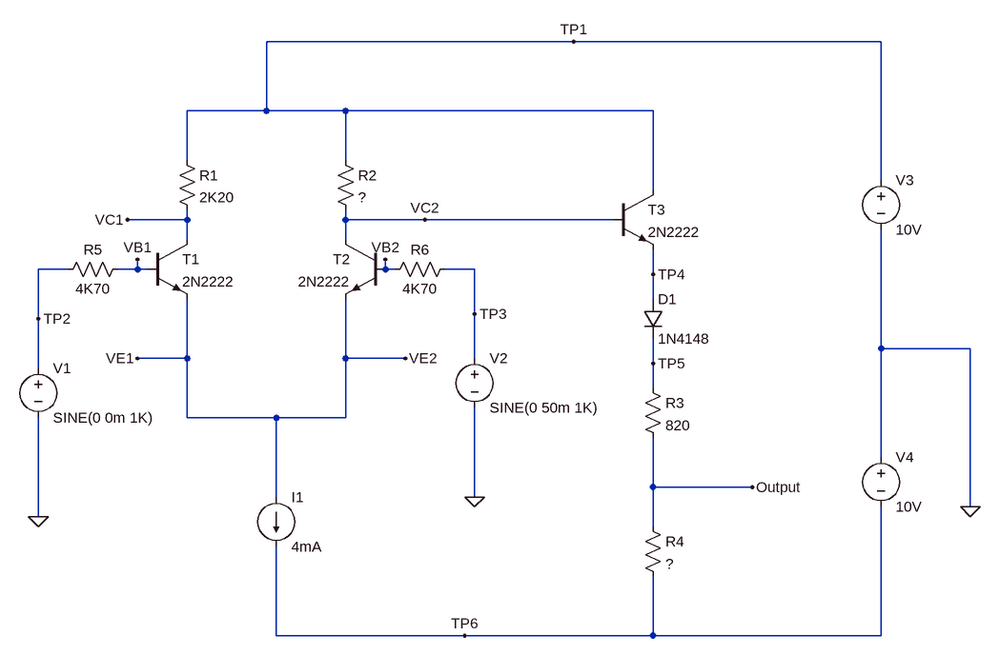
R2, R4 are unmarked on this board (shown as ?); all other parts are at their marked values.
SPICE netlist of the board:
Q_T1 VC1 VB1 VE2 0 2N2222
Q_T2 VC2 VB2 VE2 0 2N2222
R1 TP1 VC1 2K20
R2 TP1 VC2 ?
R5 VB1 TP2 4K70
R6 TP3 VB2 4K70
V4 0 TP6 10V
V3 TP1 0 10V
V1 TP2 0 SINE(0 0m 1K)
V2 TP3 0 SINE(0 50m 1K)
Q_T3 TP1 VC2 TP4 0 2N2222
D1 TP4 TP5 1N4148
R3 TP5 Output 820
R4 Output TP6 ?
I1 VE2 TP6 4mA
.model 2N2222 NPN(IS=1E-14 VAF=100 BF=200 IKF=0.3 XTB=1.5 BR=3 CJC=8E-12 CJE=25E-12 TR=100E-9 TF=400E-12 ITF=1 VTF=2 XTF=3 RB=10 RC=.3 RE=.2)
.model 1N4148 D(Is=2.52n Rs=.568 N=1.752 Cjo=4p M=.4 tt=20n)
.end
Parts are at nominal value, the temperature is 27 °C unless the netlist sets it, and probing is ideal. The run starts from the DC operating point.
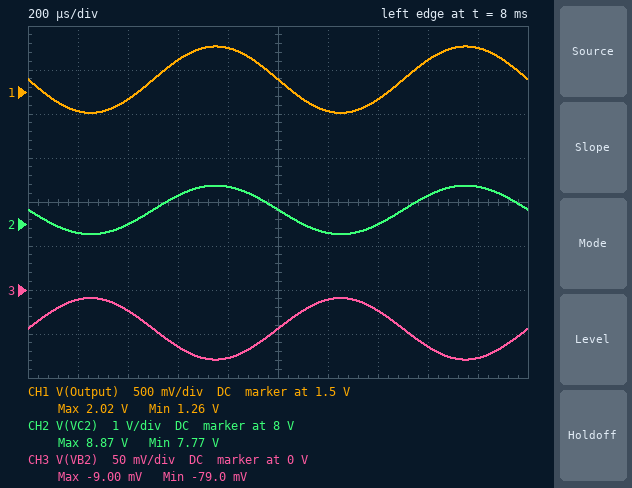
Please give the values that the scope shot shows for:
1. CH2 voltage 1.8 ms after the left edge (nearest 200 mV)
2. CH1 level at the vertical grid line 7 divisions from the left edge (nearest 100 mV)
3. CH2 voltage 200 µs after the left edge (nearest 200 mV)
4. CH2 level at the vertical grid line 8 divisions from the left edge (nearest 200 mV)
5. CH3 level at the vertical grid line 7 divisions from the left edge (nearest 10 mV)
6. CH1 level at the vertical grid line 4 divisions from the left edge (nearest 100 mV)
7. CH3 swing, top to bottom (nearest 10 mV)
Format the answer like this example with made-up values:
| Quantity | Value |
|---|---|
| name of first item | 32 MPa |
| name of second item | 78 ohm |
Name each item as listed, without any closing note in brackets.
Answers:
| Quantity | Value |
|---|---|
| CH2 voltage 1.8 ms after the left edge | 8.8 V |
| CH1 level at the vertical grid line 7 divisions from the left edge | 1.4 V |
| CH2 voltage 200 µs after the left edge | 7.8 V |
| CH2 level at the vertical grid line 8 divisions from the left edge | 8.6 V |
| CH3 level at the vertical grid line 7 divisions from the left edge | -20 mV |
| CH1 level at the vertical grid line 4 divisions from the left edge | 2.0 V |
| CH3 swing, top to bottom | 70 mV |
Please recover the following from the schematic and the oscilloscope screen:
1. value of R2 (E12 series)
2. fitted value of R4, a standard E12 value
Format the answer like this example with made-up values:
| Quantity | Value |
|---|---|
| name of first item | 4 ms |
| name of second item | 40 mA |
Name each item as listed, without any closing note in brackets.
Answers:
| Quantity | Value |
|---|---|
| value of R2 | 820 Ω |
| fitted value of R4, a standard E12 value | 1.8 kΩ |
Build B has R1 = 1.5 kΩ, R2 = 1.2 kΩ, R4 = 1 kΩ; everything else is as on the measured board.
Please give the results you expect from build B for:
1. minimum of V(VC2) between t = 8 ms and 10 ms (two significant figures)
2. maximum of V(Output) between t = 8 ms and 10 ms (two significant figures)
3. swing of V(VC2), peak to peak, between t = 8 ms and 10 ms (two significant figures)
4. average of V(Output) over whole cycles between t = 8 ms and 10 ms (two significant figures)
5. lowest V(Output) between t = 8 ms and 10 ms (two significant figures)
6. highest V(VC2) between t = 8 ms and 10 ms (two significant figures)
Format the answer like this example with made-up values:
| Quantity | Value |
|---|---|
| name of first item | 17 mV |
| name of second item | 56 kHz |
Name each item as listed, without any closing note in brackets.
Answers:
| Quantity | Value |
|---|---|
| minimum of V(VC2) between t = 8 ms and 10 ms | 6.7 V |
| maximum of V(Output) between t = 8 ms and 10 ms | -680 mV |
| swing of V(VC2), peak to peak, between t = 8 ms and 10 ms | 1.6 V |
| average of V(Output) over whole cycles between t = 8 ms and 10 ms | -1.1 V |
| lowest V(Output) between t = 8 ms and 10 ms | -1.6 V |
| highest V(VC2) between t = 8 ms and 10 ms | 8.4 V |
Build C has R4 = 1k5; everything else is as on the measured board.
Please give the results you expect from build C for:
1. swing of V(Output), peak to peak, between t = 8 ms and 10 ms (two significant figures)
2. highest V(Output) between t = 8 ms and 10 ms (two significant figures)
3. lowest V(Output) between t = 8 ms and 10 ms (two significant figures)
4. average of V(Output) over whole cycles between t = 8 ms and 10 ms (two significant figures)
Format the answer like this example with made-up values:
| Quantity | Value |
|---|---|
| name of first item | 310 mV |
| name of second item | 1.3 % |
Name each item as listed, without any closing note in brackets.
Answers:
| Quantity | Value |
|---|---|
| swing of V(Output), peak to peak, between t = 8 ms and 10 ms | 710 mV |
| highest V(Output) between t = 8 ms and 10 ms | 1.3 V |
| lowest V(Output) between t = 8 ms and 10 ms | 590 mV |
| average of V(Output) over whole cycles between t = 8 ms and 10 ms | 950 mV |
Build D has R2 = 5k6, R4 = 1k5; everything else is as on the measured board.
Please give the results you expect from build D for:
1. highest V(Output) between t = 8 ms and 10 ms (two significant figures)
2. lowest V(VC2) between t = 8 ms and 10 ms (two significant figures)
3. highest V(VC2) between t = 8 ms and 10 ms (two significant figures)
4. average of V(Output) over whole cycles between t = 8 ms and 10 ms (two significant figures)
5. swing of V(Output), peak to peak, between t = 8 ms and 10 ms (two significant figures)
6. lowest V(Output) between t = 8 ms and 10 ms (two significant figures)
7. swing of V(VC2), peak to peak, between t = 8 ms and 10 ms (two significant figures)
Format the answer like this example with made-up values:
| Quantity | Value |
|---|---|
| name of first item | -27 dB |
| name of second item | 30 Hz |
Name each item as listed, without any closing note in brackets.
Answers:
| Quantity | Value |
|---|---|
| highest V(Output) between t = 8 ms and 10 ms | -2.7 V |
| lowest V(VC2) between t = 8 ms and 10 ms | -610 mV |
| highest V(VC2) between t = 8 ms and 10 ms | 2.6 V |
| average of V(Output) over whole cycles between t = 8 ms and 10 ms | -4.2 V |
| swing of V(Output), peak to peak, between t = 8 ms and 10 ms | 2.1 V |
| lowest V(Output) between t = 8 ms and 10 ms | -4.8 V |
| swing of V(VC2), peak to peak, between t = 8 ms and 10 ms | 3.2 V |
